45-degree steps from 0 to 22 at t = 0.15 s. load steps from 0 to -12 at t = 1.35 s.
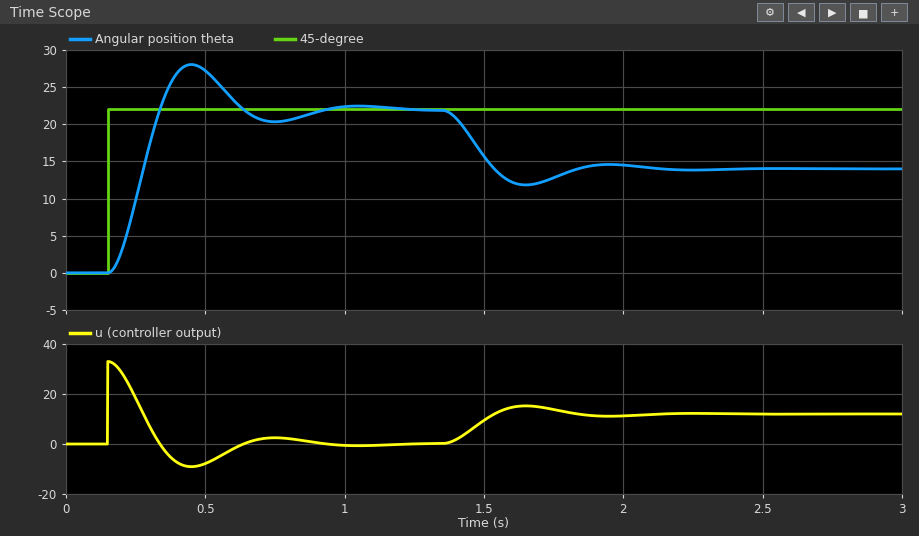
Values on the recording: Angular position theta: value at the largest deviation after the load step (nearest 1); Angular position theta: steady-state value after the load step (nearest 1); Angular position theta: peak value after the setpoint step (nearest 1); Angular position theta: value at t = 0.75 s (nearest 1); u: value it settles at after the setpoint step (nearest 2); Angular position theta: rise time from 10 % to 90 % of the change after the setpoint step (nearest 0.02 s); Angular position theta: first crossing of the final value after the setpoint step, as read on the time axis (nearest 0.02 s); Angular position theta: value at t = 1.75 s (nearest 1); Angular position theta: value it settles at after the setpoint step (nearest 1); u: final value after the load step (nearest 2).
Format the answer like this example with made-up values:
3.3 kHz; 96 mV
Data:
12; 14; 28; 20; 0; 0.12 s; 0.34 s; 13; 22; 12
